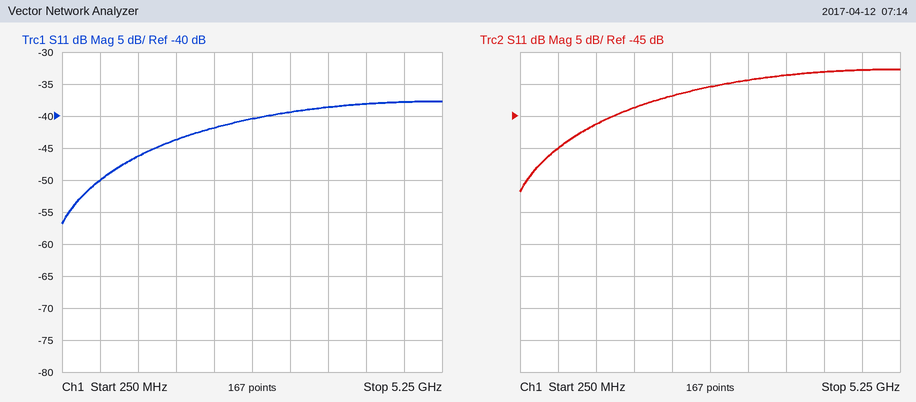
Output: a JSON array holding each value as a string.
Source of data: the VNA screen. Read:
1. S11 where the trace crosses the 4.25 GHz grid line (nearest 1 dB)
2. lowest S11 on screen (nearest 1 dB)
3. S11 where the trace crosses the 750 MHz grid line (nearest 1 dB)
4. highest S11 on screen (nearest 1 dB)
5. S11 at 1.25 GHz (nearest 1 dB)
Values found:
["-38 dB", "-57 dB", "-50 dB", "-38 dB", "-46 dB"]
